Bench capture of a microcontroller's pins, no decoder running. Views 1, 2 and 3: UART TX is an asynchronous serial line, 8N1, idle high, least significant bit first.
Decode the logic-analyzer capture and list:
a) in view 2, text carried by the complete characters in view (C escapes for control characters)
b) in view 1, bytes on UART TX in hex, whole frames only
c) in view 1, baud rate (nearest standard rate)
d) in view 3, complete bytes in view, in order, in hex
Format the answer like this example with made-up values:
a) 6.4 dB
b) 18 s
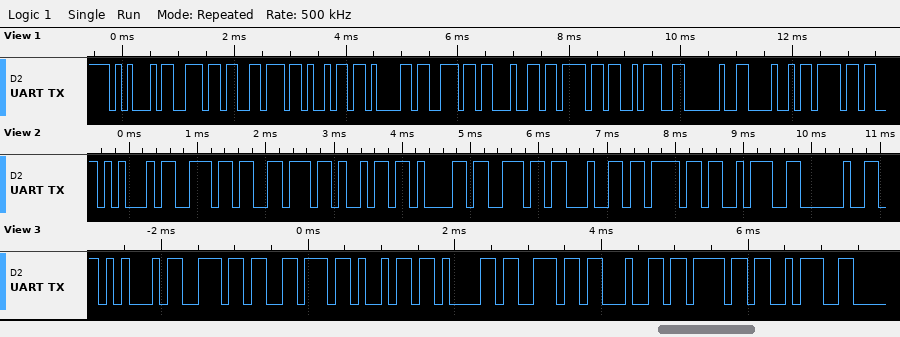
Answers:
a) "Enviando: "
b) 0x45 0x6E 0x76 0x69 0x61 0x6E 0x64 0x6F 0x3A 0x20 0x48 0x6F
c) 9600 baud
d) 45 6E 76 69 61 6E 64 6F 3A
